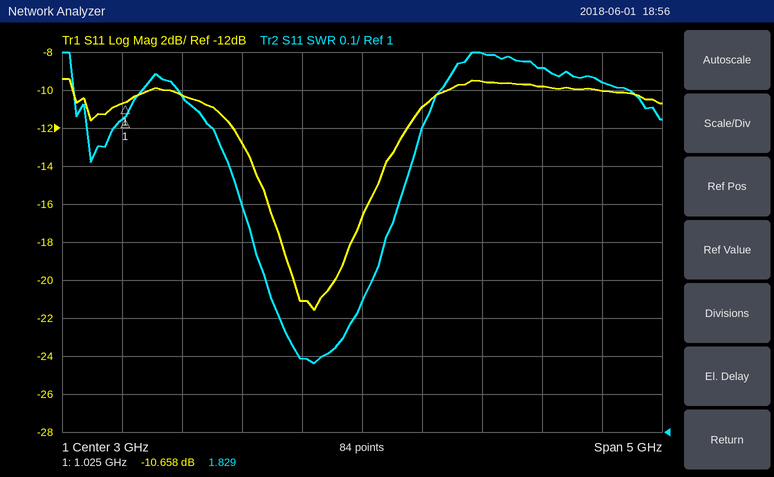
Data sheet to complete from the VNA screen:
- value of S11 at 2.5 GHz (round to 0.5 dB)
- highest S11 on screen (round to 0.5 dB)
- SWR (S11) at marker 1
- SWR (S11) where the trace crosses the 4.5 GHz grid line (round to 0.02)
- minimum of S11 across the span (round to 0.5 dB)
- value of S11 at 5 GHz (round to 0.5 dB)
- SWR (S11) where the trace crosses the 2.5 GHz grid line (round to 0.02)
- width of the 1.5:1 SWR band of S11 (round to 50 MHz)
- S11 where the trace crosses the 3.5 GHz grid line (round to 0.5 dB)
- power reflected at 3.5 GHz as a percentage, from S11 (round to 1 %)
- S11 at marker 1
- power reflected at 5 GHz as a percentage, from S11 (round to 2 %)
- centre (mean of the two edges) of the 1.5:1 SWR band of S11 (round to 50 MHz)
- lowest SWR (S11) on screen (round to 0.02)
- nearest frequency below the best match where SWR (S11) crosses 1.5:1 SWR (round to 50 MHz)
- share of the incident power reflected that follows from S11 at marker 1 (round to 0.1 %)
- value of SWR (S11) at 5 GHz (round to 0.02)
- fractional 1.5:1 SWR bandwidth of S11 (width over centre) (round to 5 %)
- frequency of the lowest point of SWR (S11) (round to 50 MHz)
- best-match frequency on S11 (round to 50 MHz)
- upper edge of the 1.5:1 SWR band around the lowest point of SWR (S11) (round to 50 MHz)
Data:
-21.0 dB
-9.5 dB
1.829
1.96
-21.5 dB
-10.0 dB
1.20
1.10 GHz
-11.0 dB
8 %
-10.658 dB
10 %
2.65 GHz
1.18
2.10 GHz
8.6 %
1.92
40 %
2.60 GHz
2.60 GHz
3.20 GHz
